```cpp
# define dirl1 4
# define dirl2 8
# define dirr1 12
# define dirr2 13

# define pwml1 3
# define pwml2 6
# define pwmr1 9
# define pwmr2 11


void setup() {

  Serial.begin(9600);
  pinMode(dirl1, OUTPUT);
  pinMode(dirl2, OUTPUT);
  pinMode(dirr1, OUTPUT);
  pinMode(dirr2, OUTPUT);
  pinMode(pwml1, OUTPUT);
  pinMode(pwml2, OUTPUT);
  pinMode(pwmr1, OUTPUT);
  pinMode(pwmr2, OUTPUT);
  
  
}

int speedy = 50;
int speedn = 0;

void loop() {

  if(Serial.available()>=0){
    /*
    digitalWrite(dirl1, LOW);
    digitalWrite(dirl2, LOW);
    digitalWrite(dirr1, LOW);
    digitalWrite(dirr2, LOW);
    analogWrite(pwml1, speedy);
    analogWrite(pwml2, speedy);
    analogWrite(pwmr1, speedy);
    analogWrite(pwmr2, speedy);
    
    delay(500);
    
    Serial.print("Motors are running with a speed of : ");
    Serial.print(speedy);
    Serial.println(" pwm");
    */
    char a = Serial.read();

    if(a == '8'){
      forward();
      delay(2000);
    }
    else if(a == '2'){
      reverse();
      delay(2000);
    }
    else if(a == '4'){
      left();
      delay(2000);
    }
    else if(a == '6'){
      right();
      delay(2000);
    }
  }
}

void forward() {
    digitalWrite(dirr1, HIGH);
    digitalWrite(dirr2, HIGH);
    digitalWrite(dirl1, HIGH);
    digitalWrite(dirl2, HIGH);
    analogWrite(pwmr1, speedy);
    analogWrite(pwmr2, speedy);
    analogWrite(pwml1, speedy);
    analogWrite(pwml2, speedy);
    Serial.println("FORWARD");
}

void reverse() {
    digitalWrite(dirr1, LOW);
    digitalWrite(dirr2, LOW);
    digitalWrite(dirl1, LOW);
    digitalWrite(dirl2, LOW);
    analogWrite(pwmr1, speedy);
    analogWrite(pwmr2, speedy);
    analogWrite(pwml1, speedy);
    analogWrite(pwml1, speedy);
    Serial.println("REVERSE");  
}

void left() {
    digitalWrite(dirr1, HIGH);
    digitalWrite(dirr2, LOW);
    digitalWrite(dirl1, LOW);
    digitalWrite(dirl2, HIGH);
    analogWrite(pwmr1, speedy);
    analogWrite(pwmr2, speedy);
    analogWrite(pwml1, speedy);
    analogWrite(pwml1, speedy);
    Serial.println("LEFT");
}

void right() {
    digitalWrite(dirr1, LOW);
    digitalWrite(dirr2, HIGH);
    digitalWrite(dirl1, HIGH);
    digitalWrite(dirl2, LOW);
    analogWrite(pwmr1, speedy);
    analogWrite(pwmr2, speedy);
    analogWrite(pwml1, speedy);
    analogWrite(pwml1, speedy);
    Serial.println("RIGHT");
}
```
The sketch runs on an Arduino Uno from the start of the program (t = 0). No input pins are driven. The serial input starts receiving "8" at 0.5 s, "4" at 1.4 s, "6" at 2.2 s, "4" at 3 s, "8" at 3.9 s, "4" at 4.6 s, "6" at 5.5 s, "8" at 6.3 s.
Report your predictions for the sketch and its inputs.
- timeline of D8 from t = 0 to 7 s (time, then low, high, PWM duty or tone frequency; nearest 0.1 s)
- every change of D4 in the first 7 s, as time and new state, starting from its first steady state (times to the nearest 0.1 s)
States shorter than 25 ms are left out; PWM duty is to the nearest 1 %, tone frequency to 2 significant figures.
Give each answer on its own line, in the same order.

0 s low; 0.5 s high; 4.5 s low; 6.5 s high
0 s low; 0.5 s high; 2.5 s low; 4.5 s high; 6.5 s low
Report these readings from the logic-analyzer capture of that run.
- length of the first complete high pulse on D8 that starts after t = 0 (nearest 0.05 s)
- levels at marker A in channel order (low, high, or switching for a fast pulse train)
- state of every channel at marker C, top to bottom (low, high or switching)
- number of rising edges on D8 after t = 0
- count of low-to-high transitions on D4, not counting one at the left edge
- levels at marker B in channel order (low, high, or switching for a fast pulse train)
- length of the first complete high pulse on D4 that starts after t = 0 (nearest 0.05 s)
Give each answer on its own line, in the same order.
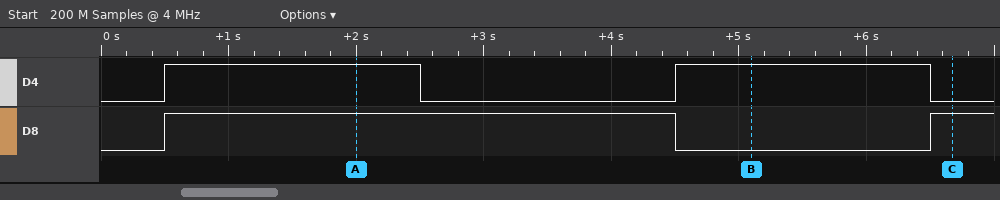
4.00 s
D4 high, D8 high
D4 low, D8 high
2
2
D4 high, D8 low
2.00 s
